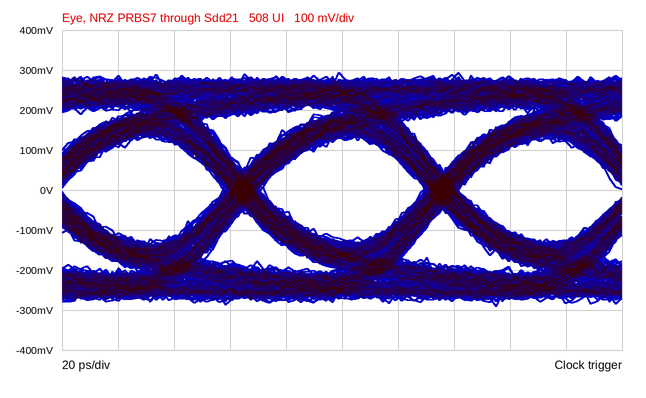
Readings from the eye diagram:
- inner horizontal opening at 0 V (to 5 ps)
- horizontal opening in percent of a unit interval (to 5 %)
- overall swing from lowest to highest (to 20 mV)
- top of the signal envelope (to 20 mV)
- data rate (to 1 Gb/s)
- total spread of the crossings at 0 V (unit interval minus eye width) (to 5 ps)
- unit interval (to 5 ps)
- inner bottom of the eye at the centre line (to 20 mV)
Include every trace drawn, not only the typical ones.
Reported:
55 ps
80 %
580 mV
300 mV
14 Gb/s
15 ps
70 ps
-120 mV
